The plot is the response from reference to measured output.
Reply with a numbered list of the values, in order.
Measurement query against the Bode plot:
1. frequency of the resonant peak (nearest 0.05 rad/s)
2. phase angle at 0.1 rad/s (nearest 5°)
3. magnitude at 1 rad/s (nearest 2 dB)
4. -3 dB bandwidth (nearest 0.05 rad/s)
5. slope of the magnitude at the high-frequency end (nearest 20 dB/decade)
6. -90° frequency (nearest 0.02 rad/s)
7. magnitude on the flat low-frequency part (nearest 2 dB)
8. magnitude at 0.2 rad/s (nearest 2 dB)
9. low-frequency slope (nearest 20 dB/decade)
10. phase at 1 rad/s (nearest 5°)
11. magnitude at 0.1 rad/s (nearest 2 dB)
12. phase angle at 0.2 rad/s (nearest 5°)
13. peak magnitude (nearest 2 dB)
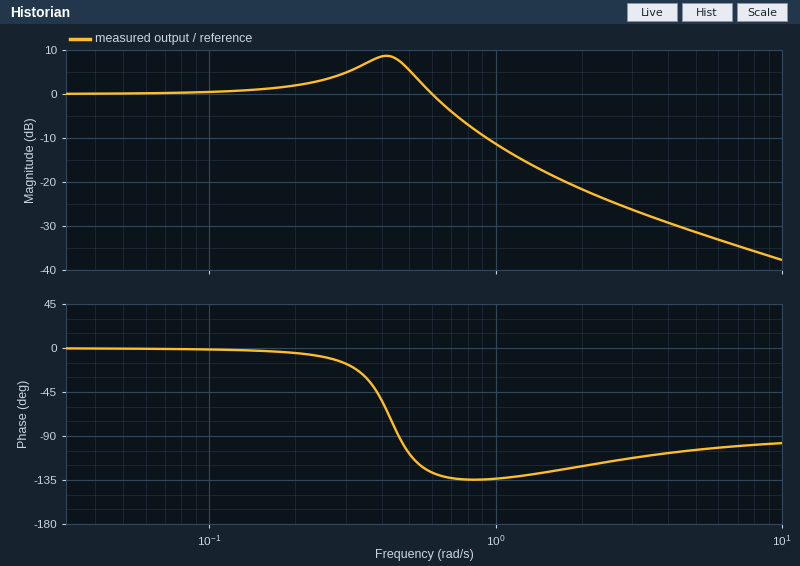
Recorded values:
1. 0.40 rad/s
2. 0°
3. -12 dB
4. 0.65 rad/s
5. -20 dB/decade
6. 0.46 rad/s
7. 0 dB
8. 2 dB
9. 0 dB/decade
10. -135°
11. 0 dB
12. -5°
13. 8 dB
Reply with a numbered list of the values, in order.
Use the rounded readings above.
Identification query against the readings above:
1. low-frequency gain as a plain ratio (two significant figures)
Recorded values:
1. 1.0
